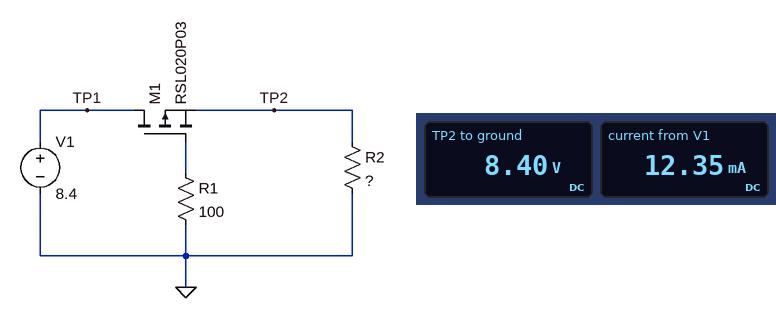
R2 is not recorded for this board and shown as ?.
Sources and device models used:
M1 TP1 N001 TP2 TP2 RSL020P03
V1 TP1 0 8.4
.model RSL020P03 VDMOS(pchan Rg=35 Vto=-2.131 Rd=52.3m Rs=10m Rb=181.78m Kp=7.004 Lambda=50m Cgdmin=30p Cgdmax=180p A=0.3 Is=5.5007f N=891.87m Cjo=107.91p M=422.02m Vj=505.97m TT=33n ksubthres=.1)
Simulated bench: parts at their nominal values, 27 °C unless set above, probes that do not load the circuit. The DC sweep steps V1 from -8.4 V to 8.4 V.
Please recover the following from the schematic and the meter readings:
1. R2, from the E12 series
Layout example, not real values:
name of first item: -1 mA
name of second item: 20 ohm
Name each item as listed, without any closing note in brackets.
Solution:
R2, from the E12 series: 680 Ω
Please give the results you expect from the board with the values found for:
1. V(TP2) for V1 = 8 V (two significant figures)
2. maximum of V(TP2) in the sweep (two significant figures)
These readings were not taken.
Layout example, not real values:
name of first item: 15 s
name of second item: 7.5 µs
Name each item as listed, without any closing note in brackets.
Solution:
V(TP2) for V1 = 8 V: 8.0 V
maximum of V(TP2) in the sweep: 8.4 V
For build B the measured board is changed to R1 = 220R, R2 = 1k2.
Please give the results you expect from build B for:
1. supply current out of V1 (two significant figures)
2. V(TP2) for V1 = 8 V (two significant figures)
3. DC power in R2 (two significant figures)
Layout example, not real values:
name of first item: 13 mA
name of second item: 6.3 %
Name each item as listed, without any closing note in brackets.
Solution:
supply current out of V1: 7.0 mA
V(TP2) for V1 = 8 V: 8.0 V
DC power in R2: 59 mW
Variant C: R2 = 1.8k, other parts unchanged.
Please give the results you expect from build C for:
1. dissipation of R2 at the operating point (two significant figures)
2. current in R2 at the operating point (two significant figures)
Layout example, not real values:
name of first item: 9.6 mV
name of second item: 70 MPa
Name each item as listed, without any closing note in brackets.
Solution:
dissipation of R2 at the operating point: 39 mW
current in R2 at the operating point: 4.7 mA
